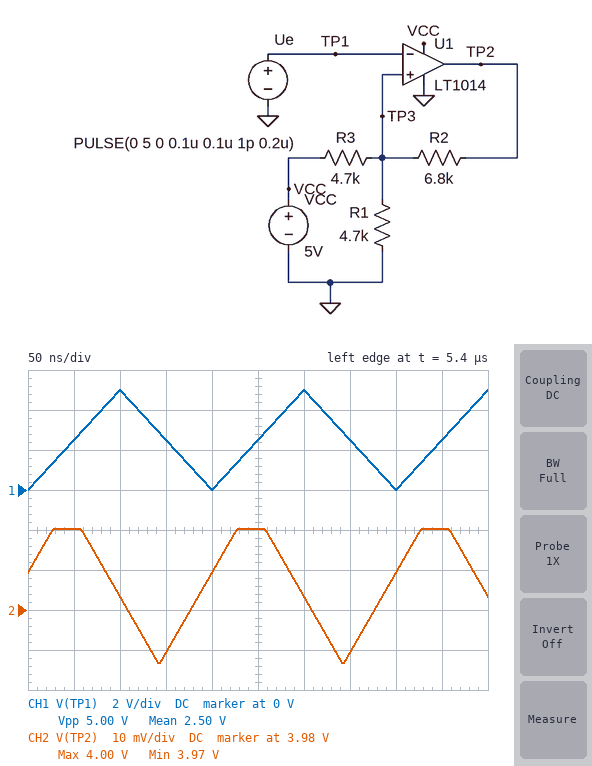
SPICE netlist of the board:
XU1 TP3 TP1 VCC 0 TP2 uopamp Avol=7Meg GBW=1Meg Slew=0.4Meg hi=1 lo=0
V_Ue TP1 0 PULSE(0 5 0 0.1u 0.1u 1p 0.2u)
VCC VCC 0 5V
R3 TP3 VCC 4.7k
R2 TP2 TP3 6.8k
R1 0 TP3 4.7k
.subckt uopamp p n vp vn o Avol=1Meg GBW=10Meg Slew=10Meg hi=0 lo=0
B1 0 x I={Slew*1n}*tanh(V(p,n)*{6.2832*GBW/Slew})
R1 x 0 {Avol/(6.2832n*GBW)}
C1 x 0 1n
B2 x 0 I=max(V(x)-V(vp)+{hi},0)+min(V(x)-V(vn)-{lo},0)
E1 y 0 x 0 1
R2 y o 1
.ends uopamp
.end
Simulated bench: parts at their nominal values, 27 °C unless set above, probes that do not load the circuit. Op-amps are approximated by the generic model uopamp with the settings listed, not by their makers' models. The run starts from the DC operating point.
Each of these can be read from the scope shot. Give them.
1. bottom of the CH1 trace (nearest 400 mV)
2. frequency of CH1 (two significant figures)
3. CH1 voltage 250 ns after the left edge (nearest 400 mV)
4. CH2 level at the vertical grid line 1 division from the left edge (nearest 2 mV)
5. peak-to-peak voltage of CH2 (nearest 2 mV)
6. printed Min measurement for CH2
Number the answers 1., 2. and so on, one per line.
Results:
1. 0 V
2. 5.0 MHz
3. 2.4 V
4. 4.000 V
5. 34 mV
6. 3.97 V
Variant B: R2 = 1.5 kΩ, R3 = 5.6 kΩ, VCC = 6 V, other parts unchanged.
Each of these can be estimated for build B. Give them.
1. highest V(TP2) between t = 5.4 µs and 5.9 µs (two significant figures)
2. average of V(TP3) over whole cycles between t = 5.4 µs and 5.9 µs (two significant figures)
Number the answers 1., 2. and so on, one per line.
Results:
1. 5.0 V
2. 4.2 V
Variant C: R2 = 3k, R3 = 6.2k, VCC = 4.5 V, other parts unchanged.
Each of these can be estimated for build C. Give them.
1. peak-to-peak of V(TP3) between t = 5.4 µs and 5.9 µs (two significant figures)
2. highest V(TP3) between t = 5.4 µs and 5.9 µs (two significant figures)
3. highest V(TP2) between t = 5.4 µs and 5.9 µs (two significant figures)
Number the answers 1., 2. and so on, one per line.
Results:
1. 17 mV
2. 2.7 V
3. 3.5 V
